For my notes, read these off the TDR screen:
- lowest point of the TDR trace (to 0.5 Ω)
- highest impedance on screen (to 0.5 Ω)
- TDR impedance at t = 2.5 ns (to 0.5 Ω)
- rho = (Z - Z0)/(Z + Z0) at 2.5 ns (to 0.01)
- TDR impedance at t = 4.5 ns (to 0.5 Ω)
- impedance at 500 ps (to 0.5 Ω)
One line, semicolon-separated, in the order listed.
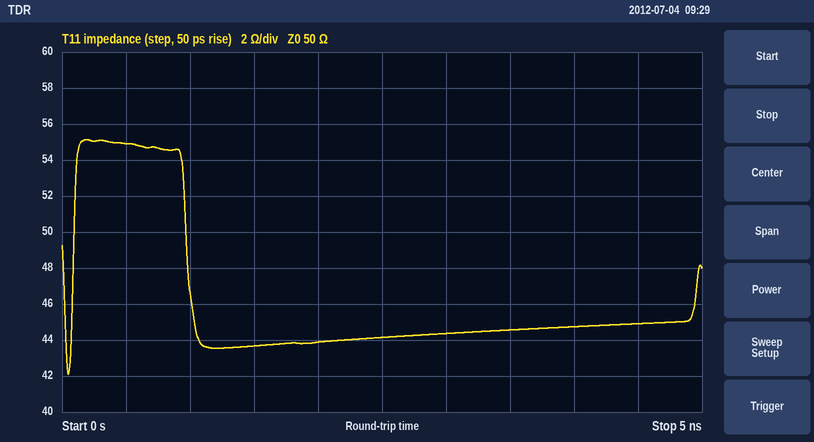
42.0 Ω; 55.0 Ω; 44.0 Ω; -0.06; 45.0 Ω; 55.0 Ω
